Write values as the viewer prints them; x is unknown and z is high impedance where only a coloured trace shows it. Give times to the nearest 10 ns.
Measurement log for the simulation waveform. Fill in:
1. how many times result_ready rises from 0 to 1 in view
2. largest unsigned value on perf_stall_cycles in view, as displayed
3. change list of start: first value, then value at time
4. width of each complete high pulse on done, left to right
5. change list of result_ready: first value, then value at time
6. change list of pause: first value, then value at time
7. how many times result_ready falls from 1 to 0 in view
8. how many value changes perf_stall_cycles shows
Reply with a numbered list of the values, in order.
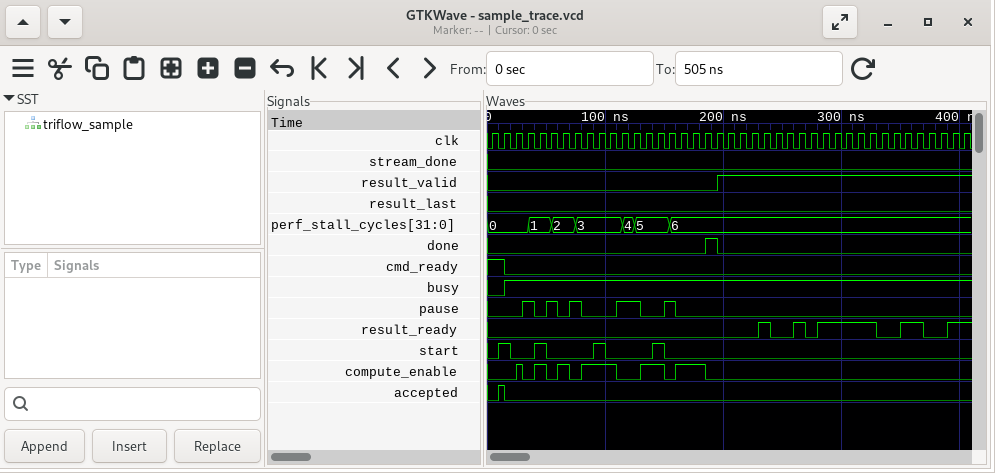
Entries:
1. 5
2. 6
3. 0, 1 at 10 ns, 0 at 20 ns, 1 at 40 ns, 0 at 50 ns, 1 at 90 ns, 0 at 100 ns, 1 at 140 ns, 0 at 150 ns
4. 10 ns
5. 0, 1 at 230 ns, 0 at 240 ns, 1 at 260 ns, 0 at 270 ns, 1 at 280 ns, 0 at 330 ns, 1 at 350 ns, 0 at 370 ns, 1 at 390 ns
6. 0, 1 at 30 ns, 0 at 40 ns, 1 at 50 ns, 0 at 60 ns, 1 at 70 ns, 0 at 80 ns, 1 at 110 ns, 0 at 130 ns, 1 at 150 ns, 0 at 160 ns
7. 4
8. 6
